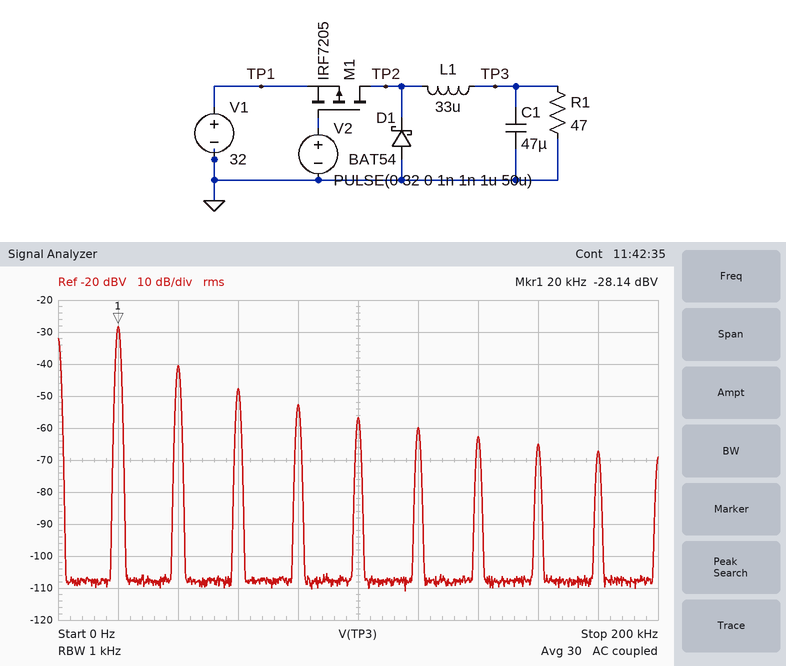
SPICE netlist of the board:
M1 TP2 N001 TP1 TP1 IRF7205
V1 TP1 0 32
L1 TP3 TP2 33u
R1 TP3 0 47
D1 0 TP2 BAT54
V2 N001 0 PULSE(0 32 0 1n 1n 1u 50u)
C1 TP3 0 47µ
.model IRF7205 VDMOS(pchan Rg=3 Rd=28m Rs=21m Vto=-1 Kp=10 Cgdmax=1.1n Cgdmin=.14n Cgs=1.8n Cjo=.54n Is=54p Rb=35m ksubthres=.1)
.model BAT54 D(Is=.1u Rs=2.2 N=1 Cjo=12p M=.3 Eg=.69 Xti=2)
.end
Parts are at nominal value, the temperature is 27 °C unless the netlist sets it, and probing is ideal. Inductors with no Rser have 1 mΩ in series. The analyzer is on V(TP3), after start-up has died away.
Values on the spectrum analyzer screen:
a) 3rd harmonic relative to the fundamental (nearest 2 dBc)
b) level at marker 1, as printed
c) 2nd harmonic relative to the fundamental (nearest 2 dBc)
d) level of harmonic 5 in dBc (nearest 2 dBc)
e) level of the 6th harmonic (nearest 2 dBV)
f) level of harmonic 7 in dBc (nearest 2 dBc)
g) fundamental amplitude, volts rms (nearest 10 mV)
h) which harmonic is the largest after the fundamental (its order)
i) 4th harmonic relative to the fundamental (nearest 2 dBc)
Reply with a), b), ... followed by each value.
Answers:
a) -20 dBc
b) -28.14 dBV
c) -12 dBc
d) -28 dBc
e) -60 dBV
f) -34 dBc
g) 40 mV
h) 2
i) -24 dBc
